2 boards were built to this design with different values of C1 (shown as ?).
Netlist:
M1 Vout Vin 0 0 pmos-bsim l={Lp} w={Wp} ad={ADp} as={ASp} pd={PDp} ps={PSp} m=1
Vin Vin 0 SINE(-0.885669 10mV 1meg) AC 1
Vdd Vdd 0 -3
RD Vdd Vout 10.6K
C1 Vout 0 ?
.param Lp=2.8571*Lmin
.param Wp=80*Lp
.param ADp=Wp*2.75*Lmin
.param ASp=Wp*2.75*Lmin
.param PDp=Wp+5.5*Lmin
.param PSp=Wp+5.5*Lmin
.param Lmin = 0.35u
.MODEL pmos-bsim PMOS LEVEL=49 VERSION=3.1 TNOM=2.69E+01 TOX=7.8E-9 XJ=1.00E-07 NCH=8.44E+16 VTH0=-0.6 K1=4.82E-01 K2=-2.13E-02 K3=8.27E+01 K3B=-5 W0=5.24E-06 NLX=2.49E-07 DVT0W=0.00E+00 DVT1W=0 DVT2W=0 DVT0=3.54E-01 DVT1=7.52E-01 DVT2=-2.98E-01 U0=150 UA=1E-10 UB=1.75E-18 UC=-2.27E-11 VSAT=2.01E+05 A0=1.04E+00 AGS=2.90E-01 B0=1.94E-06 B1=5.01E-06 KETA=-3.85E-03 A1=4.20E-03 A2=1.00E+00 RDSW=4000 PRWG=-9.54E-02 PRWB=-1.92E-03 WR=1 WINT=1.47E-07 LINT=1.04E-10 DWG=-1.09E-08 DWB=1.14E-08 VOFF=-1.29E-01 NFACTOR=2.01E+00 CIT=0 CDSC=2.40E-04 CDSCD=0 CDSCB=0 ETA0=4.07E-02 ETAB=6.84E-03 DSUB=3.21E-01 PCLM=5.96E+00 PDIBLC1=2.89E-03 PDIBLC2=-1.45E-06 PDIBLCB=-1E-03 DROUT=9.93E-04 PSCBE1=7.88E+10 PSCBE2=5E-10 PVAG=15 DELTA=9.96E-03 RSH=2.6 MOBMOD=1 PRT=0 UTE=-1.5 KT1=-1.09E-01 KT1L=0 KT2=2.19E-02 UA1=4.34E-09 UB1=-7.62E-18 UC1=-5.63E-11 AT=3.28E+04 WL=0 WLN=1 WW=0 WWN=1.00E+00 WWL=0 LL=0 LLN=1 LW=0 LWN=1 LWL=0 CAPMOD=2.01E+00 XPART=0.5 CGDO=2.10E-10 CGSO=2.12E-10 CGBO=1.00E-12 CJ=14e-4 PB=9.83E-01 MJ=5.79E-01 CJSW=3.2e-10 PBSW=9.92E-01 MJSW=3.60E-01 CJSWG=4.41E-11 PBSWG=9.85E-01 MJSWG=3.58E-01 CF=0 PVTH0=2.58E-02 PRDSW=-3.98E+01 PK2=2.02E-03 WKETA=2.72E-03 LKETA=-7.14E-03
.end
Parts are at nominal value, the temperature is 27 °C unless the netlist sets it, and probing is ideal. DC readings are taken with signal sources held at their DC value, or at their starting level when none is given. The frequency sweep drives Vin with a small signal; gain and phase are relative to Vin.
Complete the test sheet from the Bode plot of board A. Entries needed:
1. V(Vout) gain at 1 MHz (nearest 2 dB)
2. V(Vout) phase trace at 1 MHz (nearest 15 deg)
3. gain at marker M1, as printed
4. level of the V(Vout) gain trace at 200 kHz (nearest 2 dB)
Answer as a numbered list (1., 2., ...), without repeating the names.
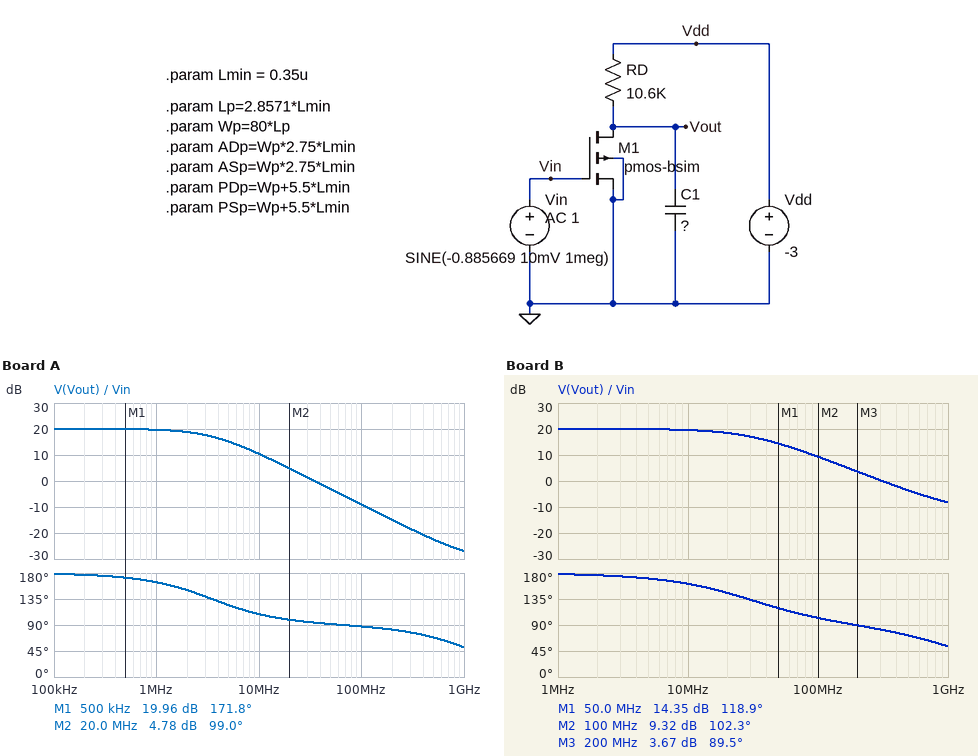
1. 20 dB
2. 165 deg
3. 19.96 dB
4. 20 dB
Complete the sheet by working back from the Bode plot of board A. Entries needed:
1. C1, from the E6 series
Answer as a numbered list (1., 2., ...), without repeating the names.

1. 4.7 pF
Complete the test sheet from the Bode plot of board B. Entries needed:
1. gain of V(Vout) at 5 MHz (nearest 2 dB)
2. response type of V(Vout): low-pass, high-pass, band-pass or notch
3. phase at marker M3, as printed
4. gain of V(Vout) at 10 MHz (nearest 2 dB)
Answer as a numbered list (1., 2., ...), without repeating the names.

1. 20 dB
2. low-pass
3. 89.5 deg
4. 20 dB
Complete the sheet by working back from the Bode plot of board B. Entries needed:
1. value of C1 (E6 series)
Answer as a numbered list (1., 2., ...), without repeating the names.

1. 470 fF
